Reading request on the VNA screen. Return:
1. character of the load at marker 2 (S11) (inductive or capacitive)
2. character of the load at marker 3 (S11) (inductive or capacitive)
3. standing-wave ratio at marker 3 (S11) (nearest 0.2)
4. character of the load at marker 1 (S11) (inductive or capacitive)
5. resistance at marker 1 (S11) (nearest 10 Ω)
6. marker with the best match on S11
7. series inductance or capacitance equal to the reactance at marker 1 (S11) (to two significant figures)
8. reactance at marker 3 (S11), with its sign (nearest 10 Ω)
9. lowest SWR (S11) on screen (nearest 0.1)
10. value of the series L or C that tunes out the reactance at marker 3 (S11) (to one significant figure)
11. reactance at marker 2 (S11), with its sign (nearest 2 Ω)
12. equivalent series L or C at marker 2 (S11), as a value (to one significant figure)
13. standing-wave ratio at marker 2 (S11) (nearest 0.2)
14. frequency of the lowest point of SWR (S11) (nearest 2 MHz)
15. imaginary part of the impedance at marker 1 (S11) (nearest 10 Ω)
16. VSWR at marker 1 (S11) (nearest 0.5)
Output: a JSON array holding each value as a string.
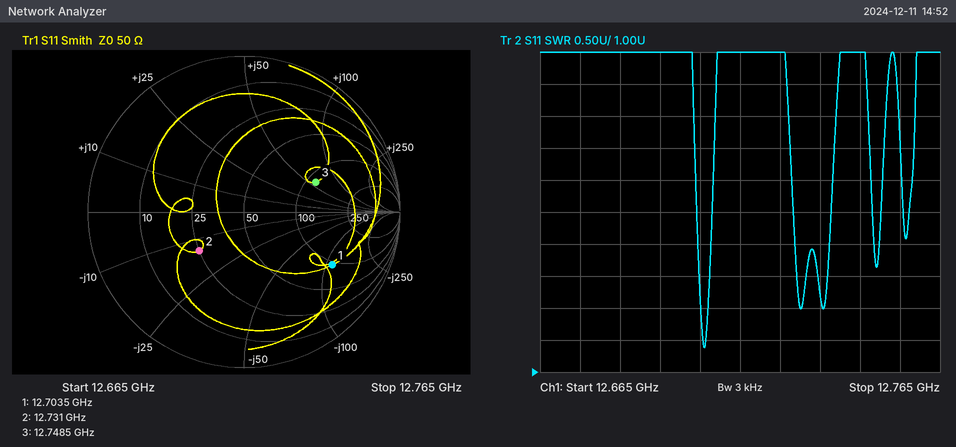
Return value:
["capacitive", "inductive", "3.0", "capacitive", "90 Ω", "marker 2", "110 fF", "+60 Ω", "1.4", "200 fF", "-14 Ω", "900 fF", "2.2", "12.706 GHz", "-110 Ω", "5.0"]
